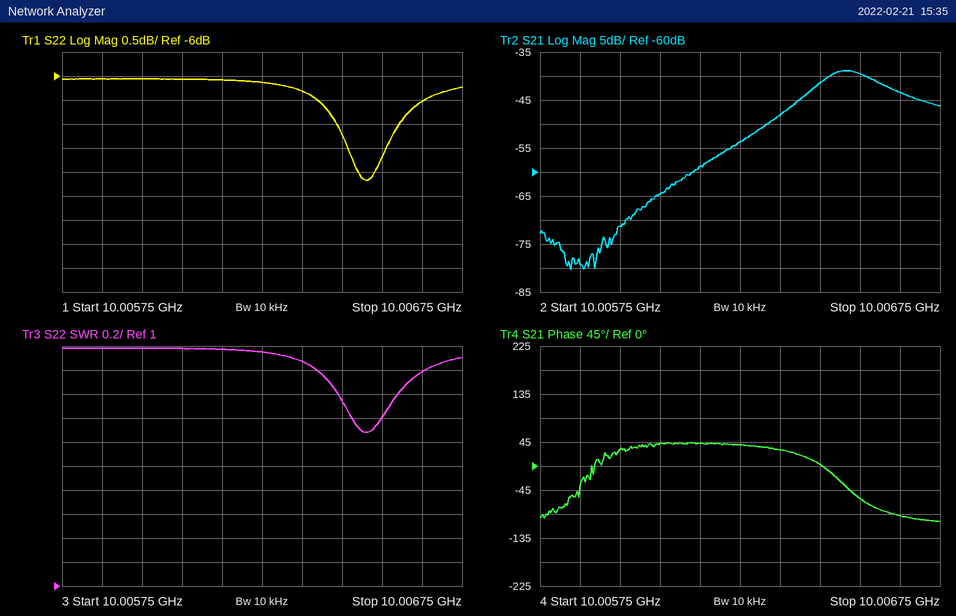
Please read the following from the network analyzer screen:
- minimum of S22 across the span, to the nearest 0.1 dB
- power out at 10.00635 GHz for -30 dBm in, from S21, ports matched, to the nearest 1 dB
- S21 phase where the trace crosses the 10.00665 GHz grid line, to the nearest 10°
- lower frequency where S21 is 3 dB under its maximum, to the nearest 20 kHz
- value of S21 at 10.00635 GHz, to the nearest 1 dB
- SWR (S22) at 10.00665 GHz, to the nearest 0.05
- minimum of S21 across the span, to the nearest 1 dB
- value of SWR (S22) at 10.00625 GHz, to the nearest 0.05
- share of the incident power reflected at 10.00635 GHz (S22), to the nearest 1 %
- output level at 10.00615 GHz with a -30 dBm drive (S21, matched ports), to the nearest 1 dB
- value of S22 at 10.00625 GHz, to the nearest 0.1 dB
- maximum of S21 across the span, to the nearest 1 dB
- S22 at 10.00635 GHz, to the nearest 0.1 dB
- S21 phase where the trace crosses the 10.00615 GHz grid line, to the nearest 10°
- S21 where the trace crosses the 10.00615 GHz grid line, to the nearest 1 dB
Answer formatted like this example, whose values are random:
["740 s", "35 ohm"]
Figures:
["-8.2 dB", "-78 dBm", "-90°", "10.00644 GHz", "-48 dB", "2.80", "-80 dB", "2.95", "23 %", "-89 dBm", "-6.1 dB", "-39 dB", "-6.3 dB", "40°", "-59 dB"]
